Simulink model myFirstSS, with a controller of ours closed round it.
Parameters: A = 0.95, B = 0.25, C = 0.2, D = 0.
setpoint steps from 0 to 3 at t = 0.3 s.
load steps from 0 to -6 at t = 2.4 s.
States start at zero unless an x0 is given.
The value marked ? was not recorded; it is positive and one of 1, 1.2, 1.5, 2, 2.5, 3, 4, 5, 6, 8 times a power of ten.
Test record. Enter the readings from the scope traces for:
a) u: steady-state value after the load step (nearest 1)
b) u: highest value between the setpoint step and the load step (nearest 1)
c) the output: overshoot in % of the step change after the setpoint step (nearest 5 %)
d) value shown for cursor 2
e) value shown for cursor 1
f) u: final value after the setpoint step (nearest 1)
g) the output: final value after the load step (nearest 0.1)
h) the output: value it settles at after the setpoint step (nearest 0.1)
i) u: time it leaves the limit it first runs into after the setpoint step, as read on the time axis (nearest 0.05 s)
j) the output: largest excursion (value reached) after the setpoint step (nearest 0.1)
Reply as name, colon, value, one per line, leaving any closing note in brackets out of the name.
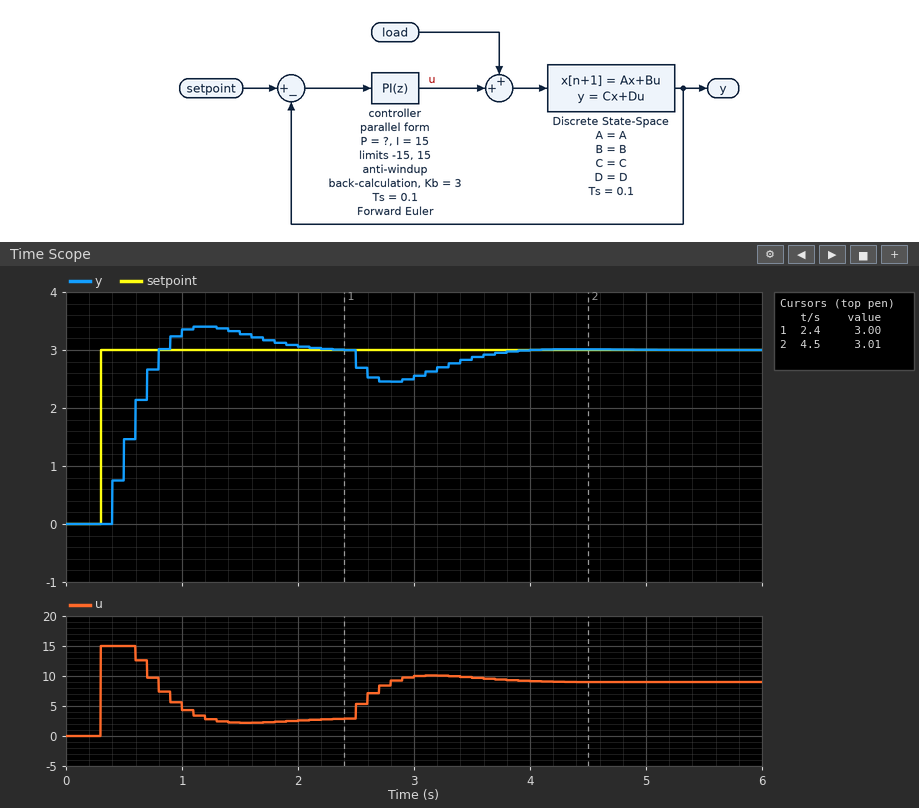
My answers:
u: steady-state value after the load step: 9
u: highest value between the setpoint step and the load step: 15
the output: overshoot in % of the step change after the setpoint step: 15 %
value shown for cursor 2: 3.01
value shown for cursor 1: 3.00
u: final value after the setpoint step: 3
the output: final value after the load step: 3.0
the output: value it settles at after the setpoint step: 3.0
u: time it leaves the limit it first runs into after the setpoint step, as read on the time axis: 0.60 s
the output: largest excursion (value reached) after the setpoint step: 3.4
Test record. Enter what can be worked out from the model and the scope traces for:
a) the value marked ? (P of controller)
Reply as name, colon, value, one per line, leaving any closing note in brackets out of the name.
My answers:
the value marked ?: 8
